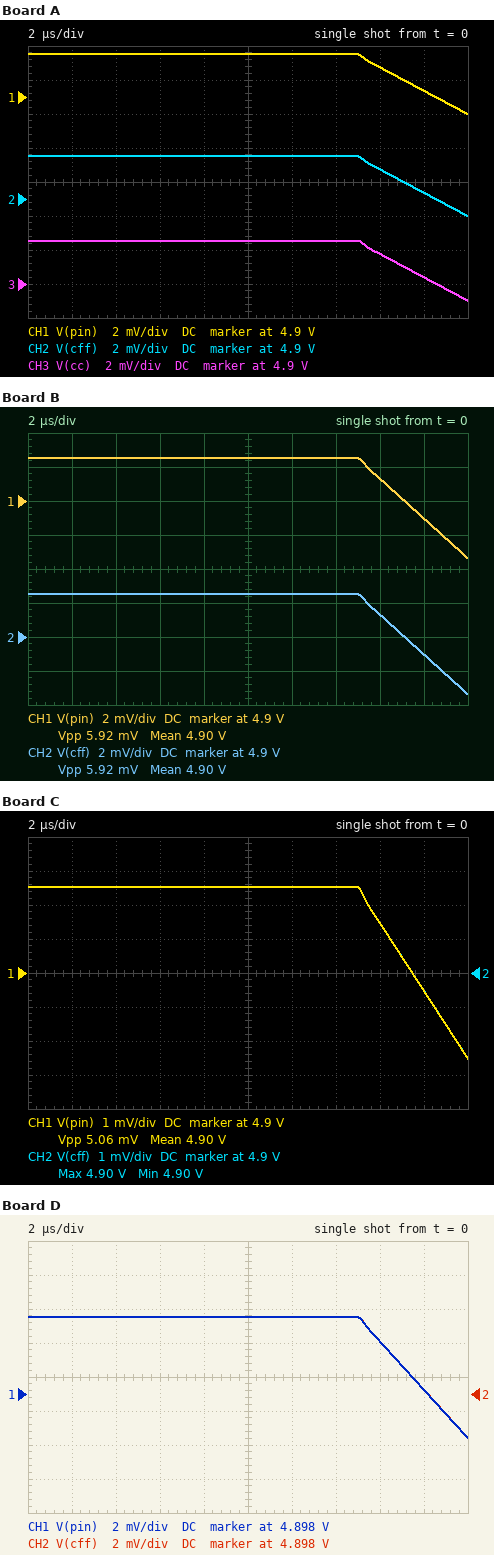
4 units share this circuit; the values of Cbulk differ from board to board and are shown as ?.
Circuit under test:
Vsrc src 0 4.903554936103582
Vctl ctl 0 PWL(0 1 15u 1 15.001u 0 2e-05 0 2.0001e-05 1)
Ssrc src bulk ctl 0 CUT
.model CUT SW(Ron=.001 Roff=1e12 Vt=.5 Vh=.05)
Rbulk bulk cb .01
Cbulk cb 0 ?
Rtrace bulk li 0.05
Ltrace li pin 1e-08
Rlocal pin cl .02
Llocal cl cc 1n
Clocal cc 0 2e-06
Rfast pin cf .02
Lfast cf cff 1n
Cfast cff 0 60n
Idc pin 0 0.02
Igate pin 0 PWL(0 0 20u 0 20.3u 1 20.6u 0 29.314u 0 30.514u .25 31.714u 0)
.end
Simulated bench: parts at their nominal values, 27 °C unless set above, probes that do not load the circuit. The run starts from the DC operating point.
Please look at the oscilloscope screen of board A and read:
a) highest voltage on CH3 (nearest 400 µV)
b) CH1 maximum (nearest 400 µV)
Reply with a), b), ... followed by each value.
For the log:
a) 4.9024 V
b) 4.9024 V
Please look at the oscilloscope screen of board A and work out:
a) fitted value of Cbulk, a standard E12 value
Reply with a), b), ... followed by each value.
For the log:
a) 27 µF
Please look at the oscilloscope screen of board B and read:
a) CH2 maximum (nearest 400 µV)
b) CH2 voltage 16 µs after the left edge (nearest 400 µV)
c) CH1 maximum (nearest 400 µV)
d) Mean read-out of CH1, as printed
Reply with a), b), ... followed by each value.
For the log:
a) 4.9024 V
b) 4.9012 V
c) 4.9024 V
d) 4.90 V
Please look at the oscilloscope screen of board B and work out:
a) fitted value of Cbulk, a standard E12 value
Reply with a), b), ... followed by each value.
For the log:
a) 15 µF
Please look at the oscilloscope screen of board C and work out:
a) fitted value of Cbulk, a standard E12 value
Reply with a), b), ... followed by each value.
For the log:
a) 18 µF
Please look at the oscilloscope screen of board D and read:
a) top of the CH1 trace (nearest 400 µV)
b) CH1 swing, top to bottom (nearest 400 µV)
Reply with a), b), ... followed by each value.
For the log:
a) 4.9024 V
b) 7.2 mV
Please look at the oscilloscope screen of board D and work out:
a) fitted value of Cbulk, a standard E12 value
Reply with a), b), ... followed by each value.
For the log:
a) 12 µF
